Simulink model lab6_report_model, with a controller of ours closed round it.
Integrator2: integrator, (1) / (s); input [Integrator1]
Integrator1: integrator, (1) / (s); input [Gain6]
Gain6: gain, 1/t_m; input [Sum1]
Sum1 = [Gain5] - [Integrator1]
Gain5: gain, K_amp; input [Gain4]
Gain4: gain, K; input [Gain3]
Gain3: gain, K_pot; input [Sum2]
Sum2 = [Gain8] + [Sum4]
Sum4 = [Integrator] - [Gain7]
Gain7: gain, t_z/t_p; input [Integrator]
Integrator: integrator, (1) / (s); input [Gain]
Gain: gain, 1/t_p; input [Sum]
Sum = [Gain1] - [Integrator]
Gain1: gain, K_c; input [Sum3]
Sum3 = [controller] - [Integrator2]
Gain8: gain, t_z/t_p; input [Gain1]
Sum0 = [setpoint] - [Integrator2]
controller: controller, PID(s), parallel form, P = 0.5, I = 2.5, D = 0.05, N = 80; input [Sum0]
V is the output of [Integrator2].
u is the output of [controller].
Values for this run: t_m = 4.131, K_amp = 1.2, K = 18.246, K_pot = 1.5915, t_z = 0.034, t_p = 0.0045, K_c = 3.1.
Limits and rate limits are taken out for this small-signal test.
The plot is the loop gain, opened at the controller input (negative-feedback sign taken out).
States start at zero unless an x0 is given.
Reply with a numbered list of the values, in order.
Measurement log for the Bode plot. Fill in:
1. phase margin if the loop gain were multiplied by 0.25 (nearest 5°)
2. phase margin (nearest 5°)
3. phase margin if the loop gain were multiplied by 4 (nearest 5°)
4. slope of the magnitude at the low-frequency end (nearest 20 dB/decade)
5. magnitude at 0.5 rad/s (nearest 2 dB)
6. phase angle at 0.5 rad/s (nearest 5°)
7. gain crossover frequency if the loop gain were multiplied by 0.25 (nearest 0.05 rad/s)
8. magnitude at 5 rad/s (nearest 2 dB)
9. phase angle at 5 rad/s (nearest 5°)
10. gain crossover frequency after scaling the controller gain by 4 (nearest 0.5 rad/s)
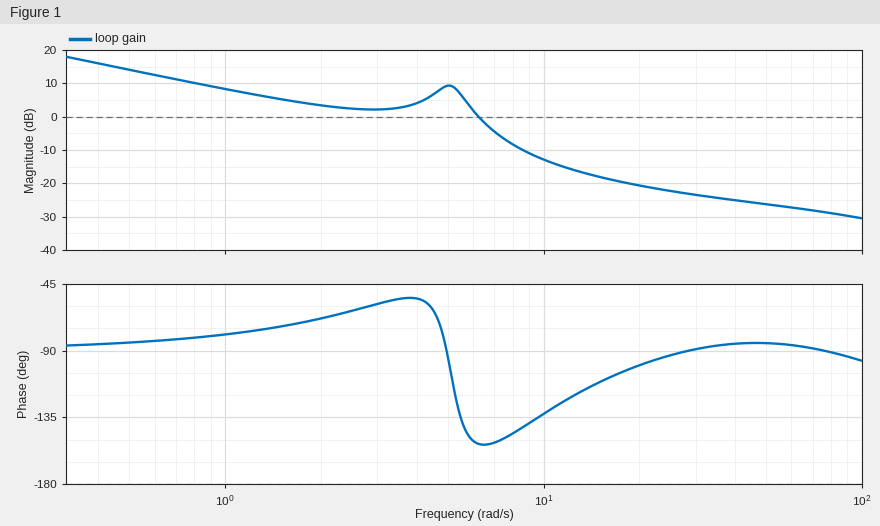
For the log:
1. 95°
2. 25°
3. 45°
4. -20 dB/decade
5. 14 dB
6. -85°
7. 0.65 rad/s
8. 10 dB
9. -95°
10. 9.5 rad/s
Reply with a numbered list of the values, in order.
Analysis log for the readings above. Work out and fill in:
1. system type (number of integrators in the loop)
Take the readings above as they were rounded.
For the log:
1. 1
